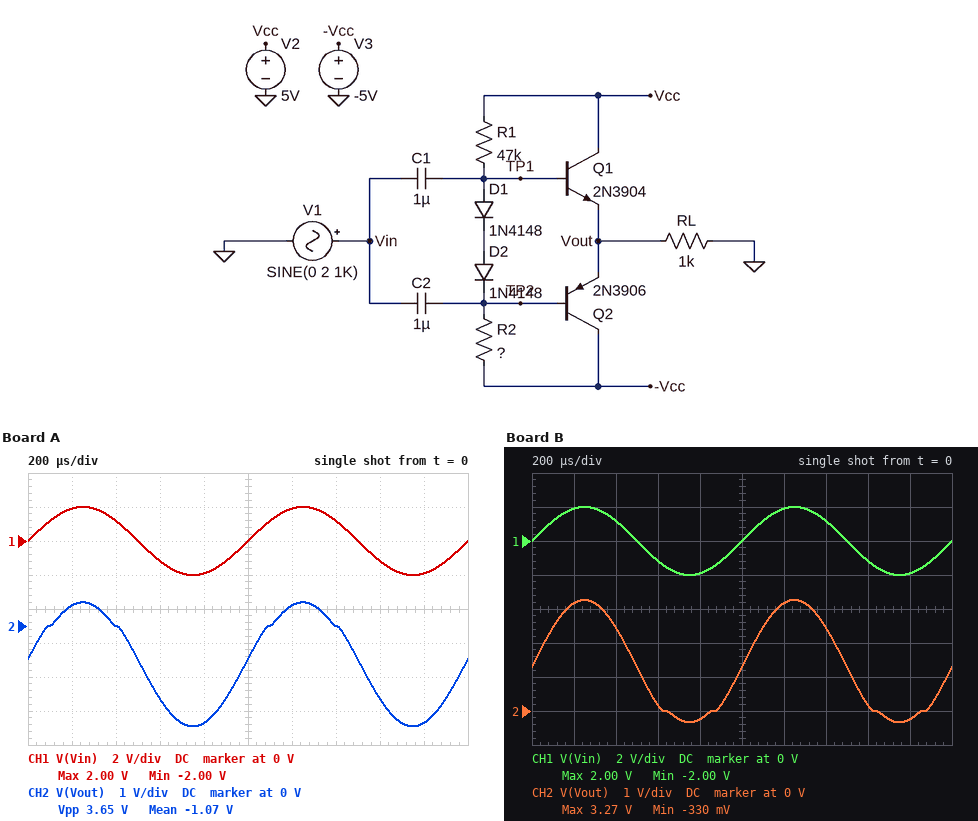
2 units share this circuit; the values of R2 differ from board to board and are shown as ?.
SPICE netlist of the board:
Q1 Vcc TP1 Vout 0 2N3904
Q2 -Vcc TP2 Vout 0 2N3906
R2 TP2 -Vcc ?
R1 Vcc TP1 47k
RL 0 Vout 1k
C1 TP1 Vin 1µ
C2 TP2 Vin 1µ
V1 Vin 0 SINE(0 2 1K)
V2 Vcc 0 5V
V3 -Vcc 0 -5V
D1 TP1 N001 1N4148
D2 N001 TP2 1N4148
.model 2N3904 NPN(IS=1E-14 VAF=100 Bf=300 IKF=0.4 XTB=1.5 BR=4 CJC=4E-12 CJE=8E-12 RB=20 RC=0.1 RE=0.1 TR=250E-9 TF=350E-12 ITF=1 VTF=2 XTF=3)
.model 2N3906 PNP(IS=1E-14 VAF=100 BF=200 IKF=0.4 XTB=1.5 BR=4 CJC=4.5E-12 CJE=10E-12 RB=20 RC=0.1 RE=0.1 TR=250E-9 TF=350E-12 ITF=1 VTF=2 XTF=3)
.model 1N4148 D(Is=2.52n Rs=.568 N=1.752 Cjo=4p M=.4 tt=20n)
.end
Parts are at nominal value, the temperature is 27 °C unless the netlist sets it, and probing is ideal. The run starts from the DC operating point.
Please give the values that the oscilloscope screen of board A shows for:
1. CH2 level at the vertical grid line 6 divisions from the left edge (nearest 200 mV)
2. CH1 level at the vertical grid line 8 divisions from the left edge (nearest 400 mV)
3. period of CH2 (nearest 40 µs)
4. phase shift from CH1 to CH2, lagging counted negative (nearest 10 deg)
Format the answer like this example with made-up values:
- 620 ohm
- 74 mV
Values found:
- 600 mV
- -1.2 V
- 1.00 ms
- 0 deg
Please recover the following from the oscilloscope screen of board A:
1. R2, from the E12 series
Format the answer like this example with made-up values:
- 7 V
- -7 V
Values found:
- 27 kΩ
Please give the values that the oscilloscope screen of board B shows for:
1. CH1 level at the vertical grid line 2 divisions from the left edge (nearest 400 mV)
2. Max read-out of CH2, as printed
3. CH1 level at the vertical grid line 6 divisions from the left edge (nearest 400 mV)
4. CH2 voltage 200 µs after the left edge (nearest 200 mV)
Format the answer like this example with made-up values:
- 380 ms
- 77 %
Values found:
- 1.2 V
- 3.27 V
- 2.0 V
- 3.2 V
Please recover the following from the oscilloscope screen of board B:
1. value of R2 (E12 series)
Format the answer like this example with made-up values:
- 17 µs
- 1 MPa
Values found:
- 100 kΩ
